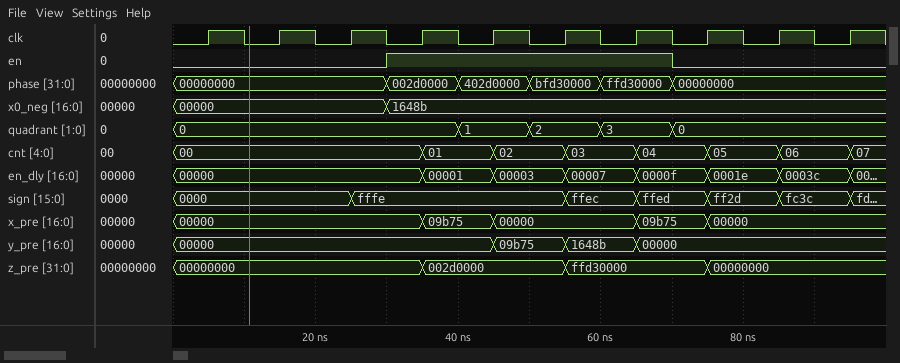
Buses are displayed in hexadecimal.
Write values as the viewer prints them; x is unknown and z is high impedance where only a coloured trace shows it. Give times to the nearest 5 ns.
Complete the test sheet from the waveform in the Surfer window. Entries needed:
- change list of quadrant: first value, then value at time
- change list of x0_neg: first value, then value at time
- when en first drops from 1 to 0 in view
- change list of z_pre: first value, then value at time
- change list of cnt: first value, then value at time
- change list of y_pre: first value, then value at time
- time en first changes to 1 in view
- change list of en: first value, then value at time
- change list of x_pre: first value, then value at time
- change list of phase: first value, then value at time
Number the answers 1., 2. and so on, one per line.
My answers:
1. 0, 1 at 40 ns, 2 at 50 ns, 3 at 60 ns, 0 at 70 ns
2. 00000, 1648b at 30 ns
3. 70 ns
4. 00000000, 002d0000 at 35 ns, ffd30000 at 55 ns, 00000000 at 75 ns
5. 00, 01 at 35 ns, 02 at 45 ns, 03 at 55 ns, 04 at 65 ns, 05 at 75 ns, 06 at 85 ns, 07 at 95 ns
6. 00000, 09b75 at 45 ns, 1648b at 55 ns, 00000 at 65 ns
7. 30 ns
8. 0, 1 at 30 ns, 0 at 70 ns
9. 00000, 09b75 at 35 ns, 00000 at 45 ns, 09b75 at 65 ns, 00000 at 75 ns
10. 00000000, 002d0000 at 30 ns, 402d0000 at 40 ns, bfd30000 at 50 ns, ffd30000 at 60 ns, 00000000 at 70 ns
